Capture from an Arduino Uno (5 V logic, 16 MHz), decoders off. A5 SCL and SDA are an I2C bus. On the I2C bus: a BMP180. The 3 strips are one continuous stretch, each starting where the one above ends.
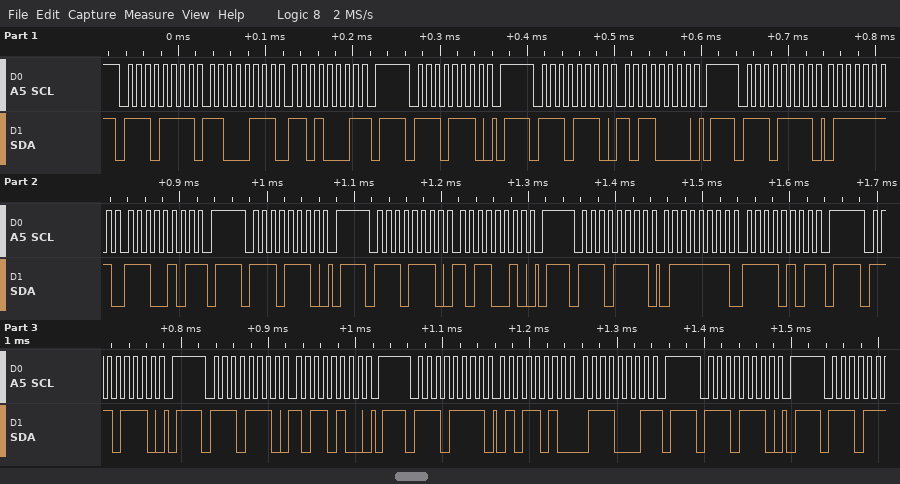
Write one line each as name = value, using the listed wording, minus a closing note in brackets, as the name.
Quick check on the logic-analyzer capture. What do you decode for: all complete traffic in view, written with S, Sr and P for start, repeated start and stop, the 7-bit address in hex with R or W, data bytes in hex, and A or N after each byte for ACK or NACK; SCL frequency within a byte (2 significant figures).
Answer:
all complete traffic in view, written with S, Sr and P for start, repeated start and stop, the 7-bit address in hex with R or W, data bytes in hex, and A or N after each byte for ACK or NACK = S 77R A C7 A D1 N P S 77W A P S 77W A B0 A P S 77R A 7F A E5 N P S 77W A P S 77W A B2 A P S 77R A 7F A F5 N P S 77W A P S 77W A B4 A P S 77R A 5A A 71 N P S 77W A P
SCL frequency within a byte = 100 kHz
